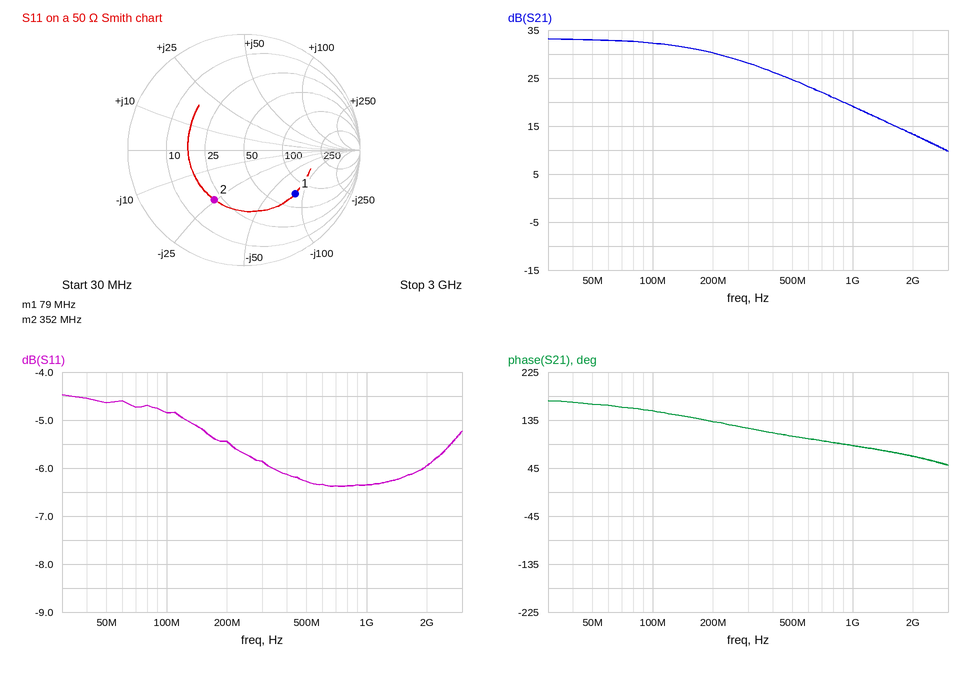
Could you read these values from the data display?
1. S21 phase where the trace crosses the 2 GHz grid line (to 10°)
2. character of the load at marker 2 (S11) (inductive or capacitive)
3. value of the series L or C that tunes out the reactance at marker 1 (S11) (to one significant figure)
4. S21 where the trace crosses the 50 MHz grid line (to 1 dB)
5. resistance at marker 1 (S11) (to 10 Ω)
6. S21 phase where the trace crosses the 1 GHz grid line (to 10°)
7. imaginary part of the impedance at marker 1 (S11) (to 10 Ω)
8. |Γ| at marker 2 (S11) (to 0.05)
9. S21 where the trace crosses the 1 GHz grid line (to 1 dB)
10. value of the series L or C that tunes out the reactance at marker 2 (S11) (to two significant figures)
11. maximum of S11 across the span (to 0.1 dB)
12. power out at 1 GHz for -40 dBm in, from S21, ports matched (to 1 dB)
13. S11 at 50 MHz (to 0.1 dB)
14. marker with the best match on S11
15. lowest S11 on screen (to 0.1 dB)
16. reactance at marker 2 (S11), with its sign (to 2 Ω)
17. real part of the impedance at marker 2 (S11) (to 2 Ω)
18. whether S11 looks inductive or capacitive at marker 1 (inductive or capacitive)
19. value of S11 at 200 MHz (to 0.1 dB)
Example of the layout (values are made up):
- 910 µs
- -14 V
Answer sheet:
- 70°
- capacitive
- 200 nH
- 33 dB
- 70 Ω
- 90°
- -80 Ω
- 0.50
- 19 dB
- 11 nH
- -4.5 dB
- -21 dBm
- -4.6 dB
- marker 2
- -6.4 dB
- -24 Ω
- 22 Ω
- capacitive
- -5.4 dB
